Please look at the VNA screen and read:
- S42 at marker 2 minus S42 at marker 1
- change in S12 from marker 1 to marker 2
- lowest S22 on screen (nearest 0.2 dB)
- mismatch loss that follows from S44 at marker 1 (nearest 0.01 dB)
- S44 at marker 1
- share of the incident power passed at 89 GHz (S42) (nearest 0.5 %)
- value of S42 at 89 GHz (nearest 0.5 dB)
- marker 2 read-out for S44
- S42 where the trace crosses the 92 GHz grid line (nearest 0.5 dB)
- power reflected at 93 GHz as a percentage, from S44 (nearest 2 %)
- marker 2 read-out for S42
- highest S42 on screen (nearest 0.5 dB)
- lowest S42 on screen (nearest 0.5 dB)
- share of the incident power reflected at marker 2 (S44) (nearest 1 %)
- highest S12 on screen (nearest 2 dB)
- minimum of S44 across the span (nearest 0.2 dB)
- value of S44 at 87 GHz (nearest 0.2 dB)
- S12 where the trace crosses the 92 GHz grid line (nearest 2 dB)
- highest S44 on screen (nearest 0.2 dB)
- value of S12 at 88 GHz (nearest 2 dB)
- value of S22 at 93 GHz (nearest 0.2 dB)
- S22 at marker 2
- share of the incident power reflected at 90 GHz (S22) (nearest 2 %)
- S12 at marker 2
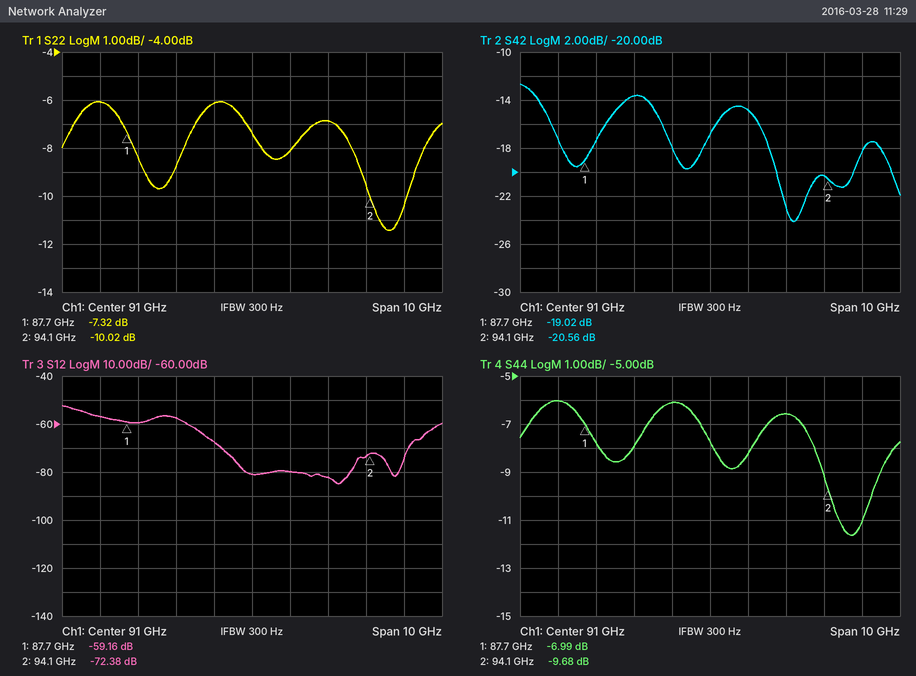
-1.54 dB
-13.22 dB
-11.4 dB
0.97 dB
-6.99 dB
4.5 %
-13.5 dB
-9.68 dB
-15.0 dB
22 %
-20.56 dB
-12.5 dB
-24.0 dB
11 %
-52 dB
-11.6 dB
-6.0 dB
-80 dB
-6.0 dB
-60 dB
-6.8 dB
-10.02 dB
24 %
-72.38 dB
